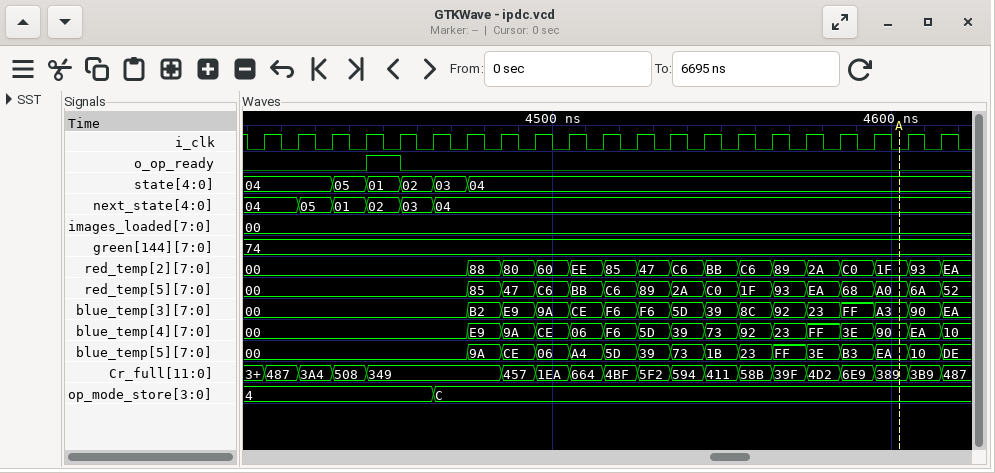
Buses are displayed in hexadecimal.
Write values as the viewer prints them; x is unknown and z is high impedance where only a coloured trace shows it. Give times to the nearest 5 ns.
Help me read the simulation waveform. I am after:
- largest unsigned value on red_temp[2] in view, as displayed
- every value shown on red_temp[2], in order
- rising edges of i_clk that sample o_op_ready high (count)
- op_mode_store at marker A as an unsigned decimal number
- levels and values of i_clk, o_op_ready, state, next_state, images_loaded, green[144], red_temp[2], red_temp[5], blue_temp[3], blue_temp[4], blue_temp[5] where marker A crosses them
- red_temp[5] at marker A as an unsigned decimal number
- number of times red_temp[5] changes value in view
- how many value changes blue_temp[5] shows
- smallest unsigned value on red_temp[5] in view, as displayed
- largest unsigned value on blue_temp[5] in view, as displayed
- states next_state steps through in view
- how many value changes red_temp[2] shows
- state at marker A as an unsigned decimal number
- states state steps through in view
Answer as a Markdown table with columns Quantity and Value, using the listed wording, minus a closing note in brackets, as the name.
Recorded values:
| Quantity | Value |
|---|---|
| largest unsigned value on red_temp[2] in view, as displayed | EE |
| every value shown on red_temp[2], in order | 00, 88, 80, 60, EE, 85, 47, C6, BB, C6, 89, 2A, C0, 1F, 93, EA |
| rising edges of i_clk that sample o_op_ready high | 1 |
| op_mode_store at marker A as an unsigned decimal number | 12 |
| levels and values of i_clk, o_op_ready, state, next_state, images_loaded, green[144], red_temp[2], red_temp[5], blue_temp[3], blue_temp[4], blue_temp[5] where marker A crosses them | i_clk=0, o_op_ready=0, state=04, next_state=04, images_loaded=00, green[144]=74, red_temp[2]=1F, red_temp[5]=A0, blue_temp[3]=A3, blue_temp[4]=90, blue_temp[5]=EA |
| red_temp[5] at marker A as an unsigned decimal number | 160 |
| number of times red_temp[5] changes value in view | 15 |
| how many value changes blue_temp[5] shows | 15 |
| smallest unsigned value on red_temp[5] in view, as displayed | 00 |
| largest unsigned value on blue_temp[5] in view, as displayed | FF |
| states next_state steps through in view | 04, 05, 01, 02, 03, 04 |
| how many value changes red_temp[2] shows | 15 |
| state at marker A as an unsigned decimal number | 4 |
| states state steps through in view | 04, 05, 01, 02, 03, 04 |
